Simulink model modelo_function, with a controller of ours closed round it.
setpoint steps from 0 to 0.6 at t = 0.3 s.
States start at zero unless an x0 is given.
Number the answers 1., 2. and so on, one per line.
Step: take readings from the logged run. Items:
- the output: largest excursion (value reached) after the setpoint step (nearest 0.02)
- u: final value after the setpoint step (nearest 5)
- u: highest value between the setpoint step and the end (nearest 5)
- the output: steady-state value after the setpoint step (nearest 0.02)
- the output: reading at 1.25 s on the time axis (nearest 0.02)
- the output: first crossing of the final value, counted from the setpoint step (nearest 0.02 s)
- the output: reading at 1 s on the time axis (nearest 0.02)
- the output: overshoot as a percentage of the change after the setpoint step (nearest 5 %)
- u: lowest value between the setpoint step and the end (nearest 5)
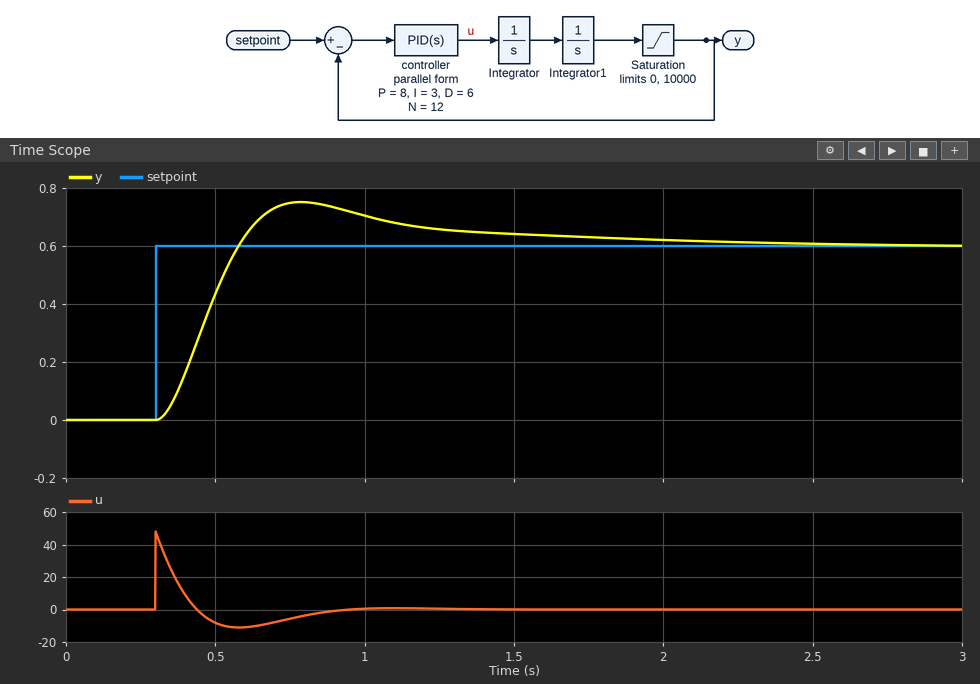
1. 0.76
2. 0
3. 50
4. 0.60
5. 0.66
6. 0.28 s
7. 0.70
8. 25 %
9. -10
